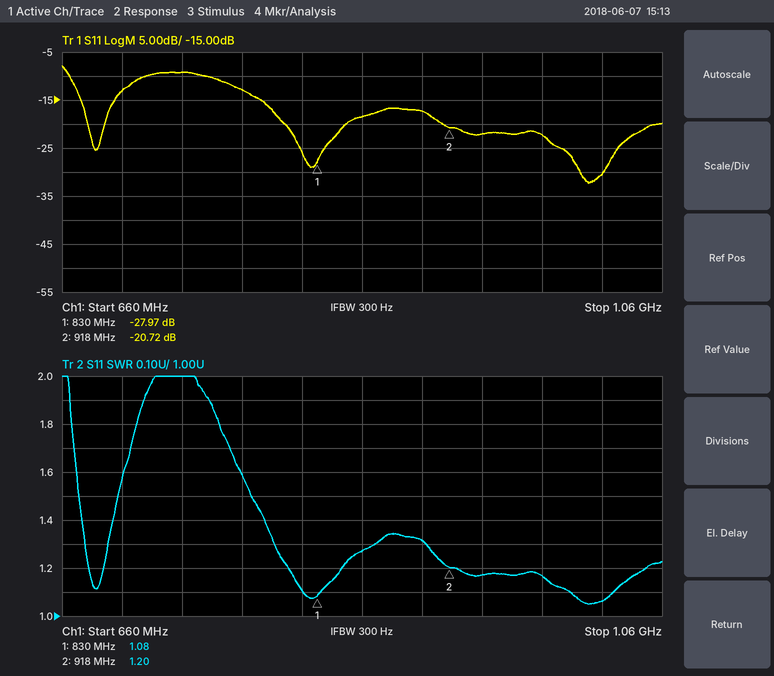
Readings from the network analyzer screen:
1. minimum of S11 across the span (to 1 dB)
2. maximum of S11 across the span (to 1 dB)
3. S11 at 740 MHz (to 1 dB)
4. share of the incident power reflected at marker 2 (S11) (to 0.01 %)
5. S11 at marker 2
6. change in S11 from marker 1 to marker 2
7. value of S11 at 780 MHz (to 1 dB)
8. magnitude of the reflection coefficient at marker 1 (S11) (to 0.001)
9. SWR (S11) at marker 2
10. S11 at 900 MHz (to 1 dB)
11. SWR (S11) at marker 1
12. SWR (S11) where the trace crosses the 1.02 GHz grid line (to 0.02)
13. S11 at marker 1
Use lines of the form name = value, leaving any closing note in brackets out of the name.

minimum of S11 across the span = -32 dB
maximum of S11 across the span = -8 dB
S11 at 740 MHz = -9 dB
share of the incident power reflected at marker 2 (S11) = 0.85 %
S11 at marker 2 = -20.72 dB
change in S11 from marker 1 to marker 2 = 7.25 dB
value of S11 at 780 MHz = -13 dB
magnitude of the reflection coefficient at marker 1 (S11) = 0.040
SWR (S11) at marker 2 = 1.20
S11 at 900 MHz = -17 dB
SWR (S11) at marker 1 = 1.08
SWR (S11) where the trace crosses the 1.02 GHz grid line = 1.06
S11 at marker 1 = -27.97 dB
